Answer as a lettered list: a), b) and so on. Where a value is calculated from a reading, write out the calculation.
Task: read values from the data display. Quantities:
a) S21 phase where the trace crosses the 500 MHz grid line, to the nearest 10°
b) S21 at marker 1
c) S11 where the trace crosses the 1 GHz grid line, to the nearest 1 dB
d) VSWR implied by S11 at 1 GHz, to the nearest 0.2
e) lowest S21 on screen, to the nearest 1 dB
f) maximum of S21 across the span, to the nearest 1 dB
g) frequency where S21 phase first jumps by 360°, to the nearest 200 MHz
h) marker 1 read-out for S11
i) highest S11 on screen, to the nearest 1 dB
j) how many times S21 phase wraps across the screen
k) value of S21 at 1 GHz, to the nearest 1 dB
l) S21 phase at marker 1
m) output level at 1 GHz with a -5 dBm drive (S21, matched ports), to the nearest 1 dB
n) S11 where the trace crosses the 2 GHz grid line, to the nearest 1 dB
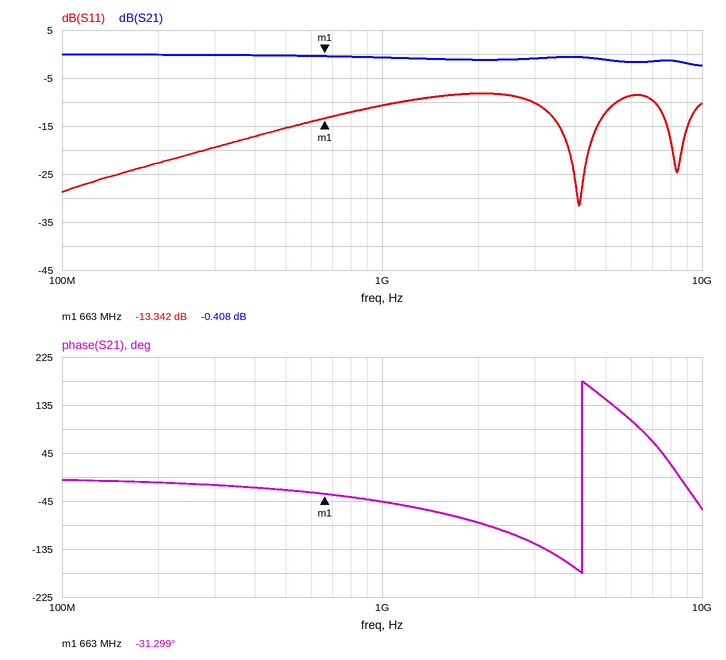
a) -20°
b) -0.408 dB
c) -11 dB
d) |Γ| = 10^(-11/20) = 0.2818; VSWR = (1 + 0.2818)/(1 − 0.2818) ≈ 1.8
e) -2 dB
f) 0 dB
g) 4.2 GHz
h) -13.342 dB
i) -8 dB
j) 1
k) -1 dB
l) -31.299°
m) -5 dBm + (-1 dB) = -6 dBm
n) -8 dB
